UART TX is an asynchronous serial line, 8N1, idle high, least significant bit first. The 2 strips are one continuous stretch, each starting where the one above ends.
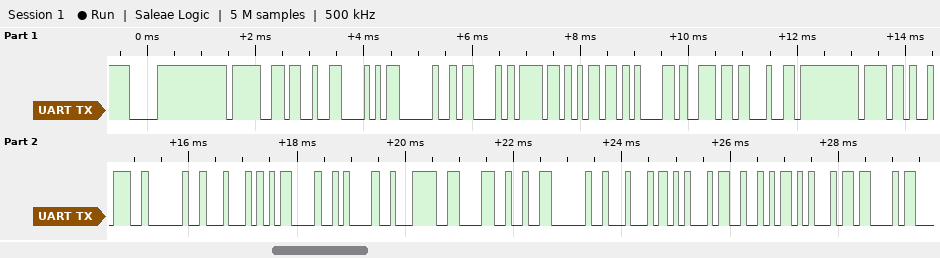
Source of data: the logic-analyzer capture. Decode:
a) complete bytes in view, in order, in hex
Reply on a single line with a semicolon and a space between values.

0xF0 0x9F 0x93 0xA8 0x20 0x43 0x6F 0x6D 0x61 0x6E 0x64 0x6F 0x3A 0x20 0x44 0x0D 0x0A 0xE2 0x86 0x92 0x20 0x44 0x45 0x52 0x45 0x43
